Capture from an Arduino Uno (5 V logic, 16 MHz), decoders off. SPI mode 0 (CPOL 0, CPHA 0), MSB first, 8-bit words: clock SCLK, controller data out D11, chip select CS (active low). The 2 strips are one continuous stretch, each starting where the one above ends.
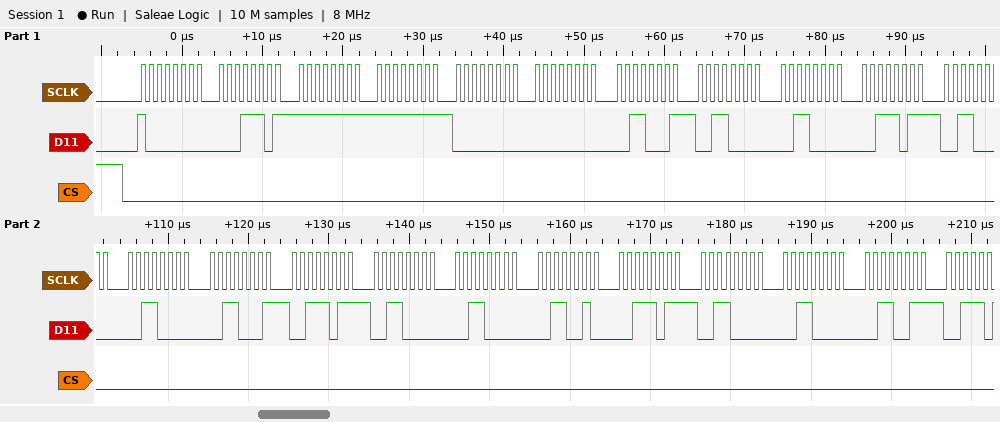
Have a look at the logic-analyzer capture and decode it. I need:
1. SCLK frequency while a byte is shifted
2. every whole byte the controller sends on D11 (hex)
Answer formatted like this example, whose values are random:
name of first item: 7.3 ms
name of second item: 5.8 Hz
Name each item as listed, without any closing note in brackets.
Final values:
SCLK frequency while a byte is shifted: 1 MHz
every whole byte the controller sends on D11: 80 1D FF FF 00 00 31 30 30 3B 30 30 31 3B 30 30 32 3B 30 30 33
